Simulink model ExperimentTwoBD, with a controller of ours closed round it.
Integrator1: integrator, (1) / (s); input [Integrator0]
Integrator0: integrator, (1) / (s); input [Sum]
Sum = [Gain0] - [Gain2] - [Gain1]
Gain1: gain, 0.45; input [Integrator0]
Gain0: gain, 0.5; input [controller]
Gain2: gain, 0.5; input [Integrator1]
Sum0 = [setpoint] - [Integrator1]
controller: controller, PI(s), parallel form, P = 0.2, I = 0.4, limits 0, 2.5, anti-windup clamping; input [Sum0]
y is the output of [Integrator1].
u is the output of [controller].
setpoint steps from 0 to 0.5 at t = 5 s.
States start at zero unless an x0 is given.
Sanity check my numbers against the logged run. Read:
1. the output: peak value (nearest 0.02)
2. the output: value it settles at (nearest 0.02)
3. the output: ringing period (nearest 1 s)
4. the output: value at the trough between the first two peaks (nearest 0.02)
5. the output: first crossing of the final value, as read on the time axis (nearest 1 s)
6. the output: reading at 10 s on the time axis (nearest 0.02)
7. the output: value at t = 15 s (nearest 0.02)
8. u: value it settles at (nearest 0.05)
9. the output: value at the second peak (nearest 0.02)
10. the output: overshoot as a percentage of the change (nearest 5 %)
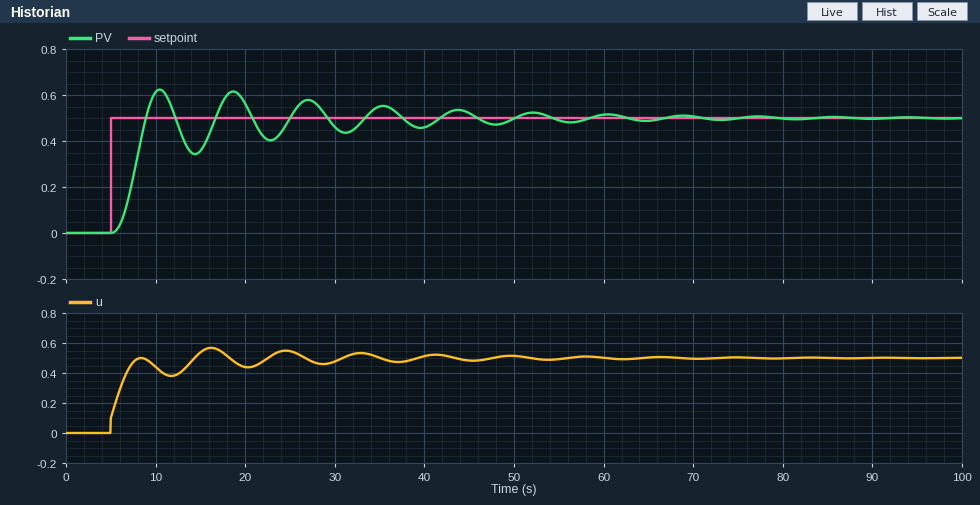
0.62
0.50
8 s
0.34
9 s
0.62
0.36
0.50
0.62
25 %
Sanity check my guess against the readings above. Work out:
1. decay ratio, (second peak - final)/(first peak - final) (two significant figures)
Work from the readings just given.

1.0
